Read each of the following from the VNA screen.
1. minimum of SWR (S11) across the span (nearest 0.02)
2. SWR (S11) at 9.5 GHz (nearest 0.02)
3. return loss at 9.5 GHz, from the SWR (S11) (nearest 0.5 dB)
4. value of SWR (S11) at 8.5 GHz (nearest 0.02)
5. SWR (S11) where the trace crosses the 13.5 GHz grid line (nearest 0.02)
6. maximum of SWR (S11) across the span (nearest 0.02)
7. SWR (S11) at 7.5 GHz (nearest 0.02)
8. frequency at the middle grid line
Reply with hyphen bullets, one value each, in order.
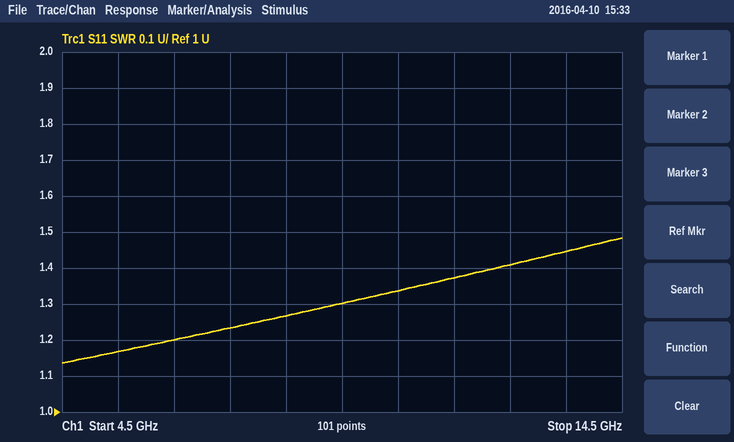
- 1.14
- 1.30
- 17.5 dB
- 1.26
- 1.44
- 1.48
- 1.24
- 9.5 GHz
